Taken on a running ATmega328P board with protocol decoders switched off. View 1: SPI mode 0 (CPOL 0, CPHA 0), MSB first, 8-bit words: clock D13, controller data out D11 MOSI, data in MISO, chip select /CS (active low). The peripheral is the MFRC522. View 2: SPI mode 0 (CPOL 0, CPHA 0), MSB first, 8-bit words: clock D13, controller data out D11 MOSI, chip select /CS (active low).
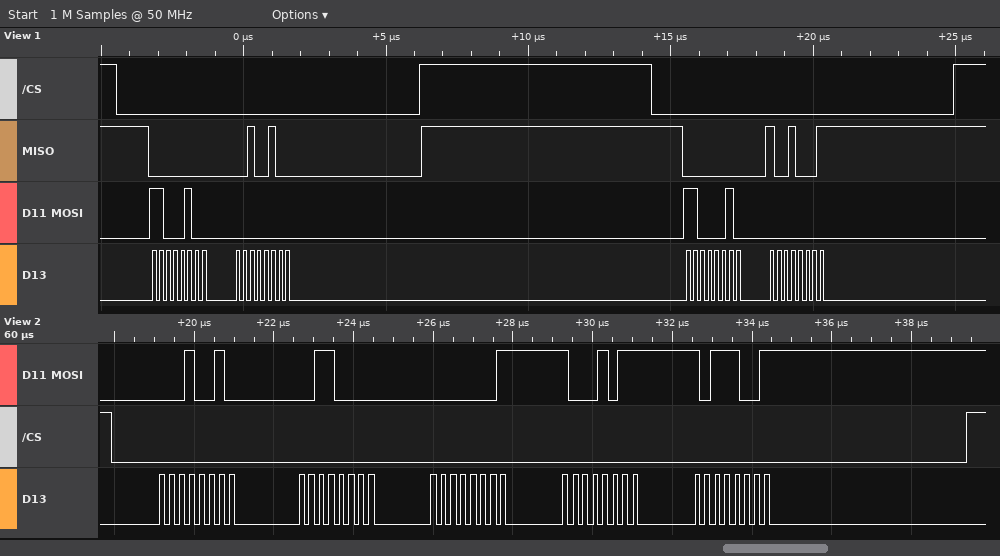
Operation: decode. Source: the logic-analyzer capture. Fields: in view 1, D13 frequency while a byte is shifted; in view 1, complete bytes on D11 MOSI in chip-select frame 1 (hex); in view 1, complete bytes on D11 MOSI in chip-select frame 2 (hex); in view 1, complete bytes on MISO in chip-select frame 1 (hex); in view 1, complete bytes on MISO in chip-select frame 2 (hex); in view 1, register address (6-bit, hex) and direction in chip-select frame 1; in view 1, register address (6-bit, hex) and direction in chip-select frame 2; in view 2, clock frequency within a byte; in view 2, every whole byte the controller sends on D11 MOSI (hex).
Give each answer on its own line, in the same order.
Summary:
4 MHz
C4 00
C2 00
00 24
00 91
0x22 read
0x21 read
4 MHz
12 30 01 8B B9
